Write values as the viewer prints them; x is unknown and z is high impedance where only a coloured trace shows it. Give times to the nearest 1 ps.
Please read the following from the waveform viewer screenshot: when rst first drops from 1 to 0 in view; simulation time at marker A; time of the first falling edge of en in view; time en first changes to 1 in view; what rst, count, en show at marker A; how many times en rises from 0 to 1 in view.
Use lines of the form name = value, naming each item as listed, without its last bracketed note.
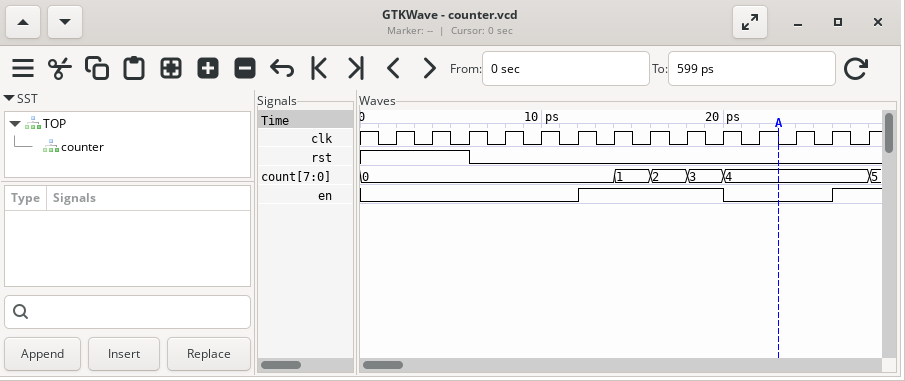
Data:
when rst first drops from 1 to 0 in view = 6 ps
simulation time at marker A = 23 ps
time of the first falling edge of en in view = 20 ps
time en first changes to 1 in view = 12 ps
what rst, count, en show at marker A = rst=0, count=4, en=0
how many times en rises from 0 to 1 in view = 2
